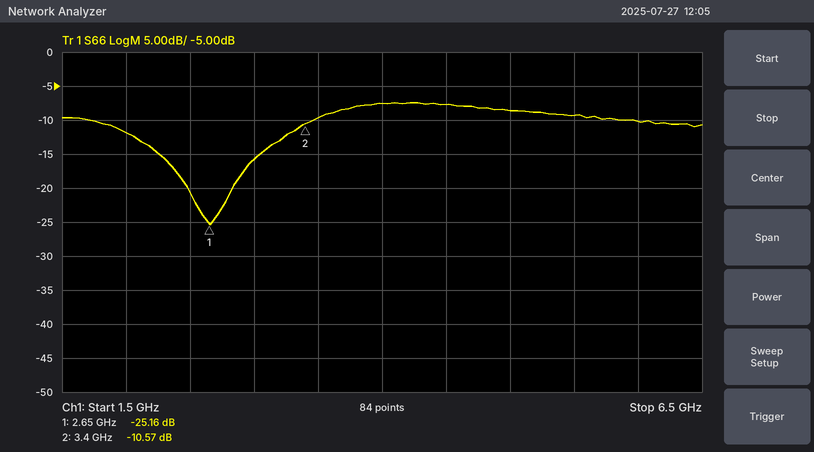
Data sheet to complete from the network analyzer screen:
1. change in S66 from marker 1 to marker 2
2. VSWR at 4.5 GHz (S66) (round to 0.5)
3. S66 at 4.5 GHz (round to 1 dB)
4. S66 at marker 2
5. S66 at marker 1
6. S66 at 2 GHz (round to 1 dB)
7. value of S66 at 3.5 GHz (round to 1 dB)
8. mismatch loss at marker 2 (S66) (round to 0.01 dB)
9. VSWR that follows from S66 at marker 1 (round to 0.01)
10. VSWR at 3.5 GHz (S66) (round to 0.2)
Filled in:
14.59 dB
2.5
-8 dB
-10.57 dB
-25.16 dB
-12 dB
-10 dB
0.40 dB
1.12
2.0
